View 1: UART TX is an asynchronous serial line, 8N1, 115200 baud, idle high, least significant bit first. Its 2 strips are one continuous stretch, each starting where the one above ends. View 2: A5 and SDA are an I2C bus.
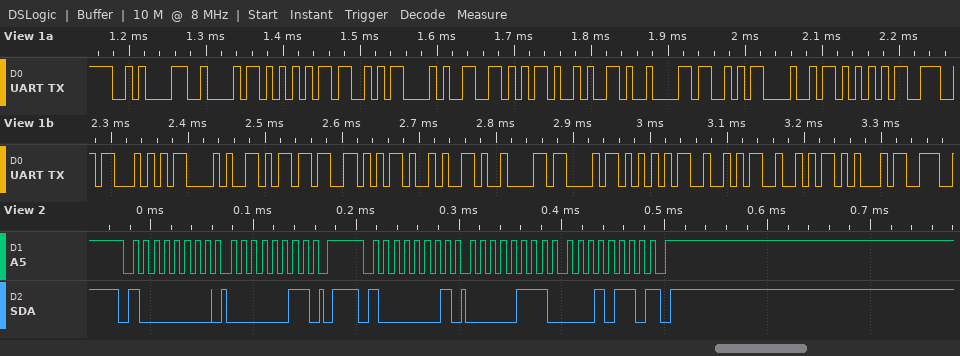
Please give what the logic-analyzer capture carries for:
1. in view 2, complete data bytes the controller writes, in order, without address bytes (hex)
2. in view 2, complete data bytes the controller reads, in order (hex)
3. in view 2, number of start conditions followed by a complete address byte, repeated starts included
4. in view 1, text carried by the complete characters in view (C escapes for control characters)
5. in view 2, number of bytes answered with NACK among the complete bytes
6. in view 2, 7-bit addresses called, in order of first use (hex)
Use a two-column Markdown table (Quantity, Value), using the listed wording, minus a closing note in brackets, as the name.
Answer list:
| Quantity | Value |
|---|---|
| in view 2, complete data bytes the controller writes, in order, without address bytes | 03 |
| in view 2, complete data bytes the controller reads, in order | 07 16 |
| in view 2, number of start conditions followed by a complete address byte, repeated starts included | 2 |
| in view 1, text carried by the complete characters in view | "\nBUS(V)\tSHUNT(mV)\tCURRE" |
| in view 2, number of bytes answered with NACK among the complete bytes | 1 |
| in view 2, 7-bit addresses called, in order of first use | 0x40 |
